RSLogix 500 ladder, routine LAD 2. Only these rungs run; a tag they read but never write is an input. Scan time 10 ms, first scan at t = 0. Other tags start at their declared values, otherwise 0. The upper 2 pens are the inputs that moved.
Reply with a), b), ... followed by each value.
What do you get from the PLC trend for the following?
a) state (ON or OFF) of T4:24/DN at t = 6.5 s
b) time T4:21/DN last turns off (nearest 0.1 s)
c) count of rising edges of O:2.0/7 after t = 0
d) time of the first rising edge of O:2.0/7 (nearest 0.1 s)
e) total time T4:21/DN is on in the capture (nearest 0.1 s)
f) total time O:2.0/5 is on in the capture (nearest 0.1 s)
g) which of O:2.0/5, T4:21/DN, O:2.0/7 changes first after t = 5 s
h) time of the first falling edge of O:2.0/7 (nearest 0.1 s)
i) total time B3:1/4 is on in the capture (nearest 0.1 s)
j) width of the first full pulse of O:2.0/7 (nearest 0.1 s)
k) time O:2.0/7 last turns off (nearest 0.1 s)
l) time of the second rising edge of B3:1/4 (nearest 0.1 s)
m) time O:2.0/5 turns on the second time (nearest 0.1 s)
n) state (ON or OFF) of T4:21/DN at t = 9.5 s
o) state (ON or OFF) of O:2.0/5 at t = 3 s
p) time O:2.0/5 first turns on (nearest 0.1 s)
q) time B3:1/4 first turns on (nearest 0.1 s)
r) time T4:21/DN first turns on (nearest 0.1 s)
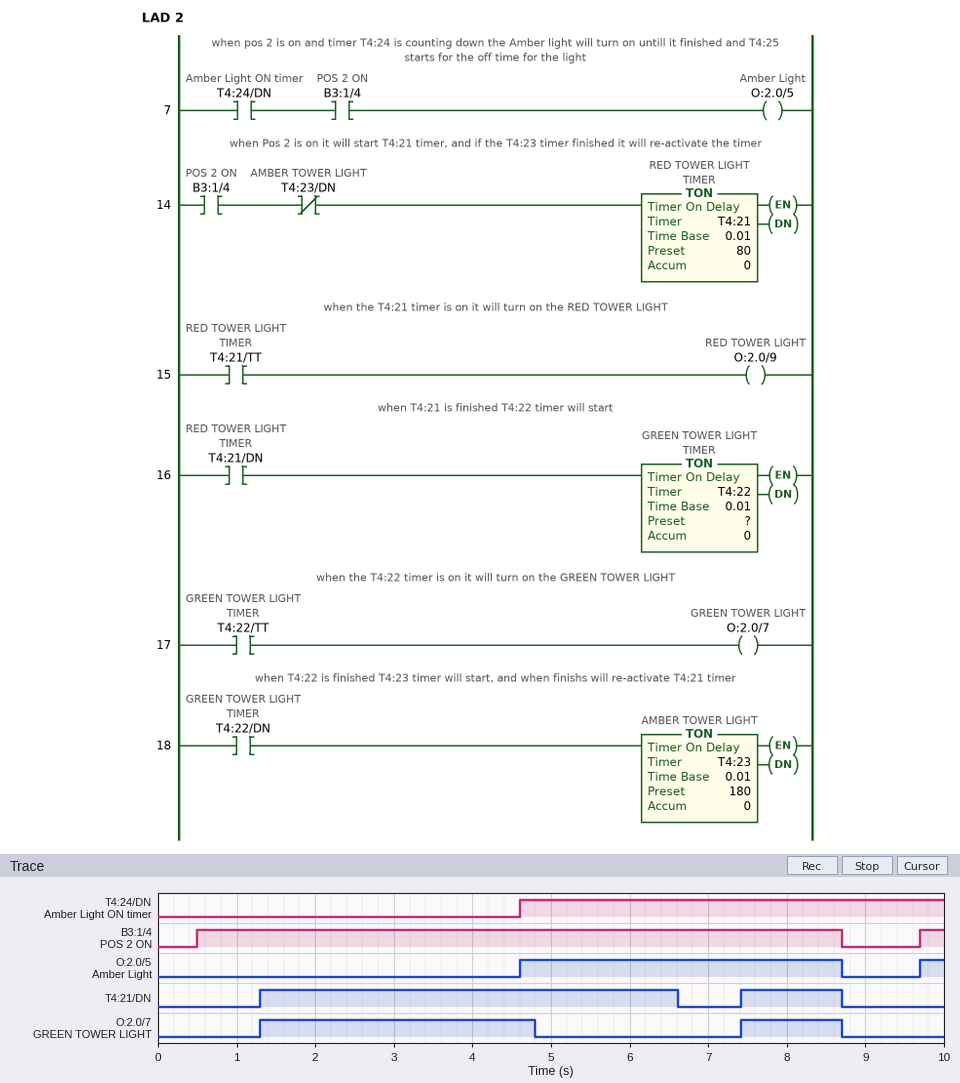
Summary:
a) ON
b) 8.7 s
c) 2
d) 1.3 s
e) 6.6 s
f) 4.4 s
g) T4:21/DN
h) 4.8 s
i) 8.5 s
j) 3.5 s
k) 8.7 s
l) 9.7 s
m) 9.7 s
n) OFF
o) OFF
p) 4.6 s
q) 0.5 s
r) 1.3 s
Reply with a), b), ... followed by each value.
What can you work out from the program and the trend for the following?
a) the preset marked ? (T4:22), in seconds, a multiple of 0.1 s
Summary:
a) 3.5 s
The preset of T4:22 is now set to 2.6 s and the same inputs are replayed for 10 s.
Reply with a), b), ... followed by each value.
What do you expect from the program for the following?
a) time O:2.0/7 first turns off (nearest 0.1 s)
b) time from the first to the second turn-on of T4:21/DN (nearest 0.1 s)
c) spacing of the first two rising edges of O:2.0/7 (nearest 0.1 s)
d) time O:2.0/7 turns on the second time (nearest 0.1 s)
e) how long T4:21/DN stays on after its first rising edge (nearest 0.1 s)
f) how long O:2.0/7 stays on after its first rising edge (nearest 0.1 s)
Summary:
a) 3.9 s
b) 5.2 s
c) 5.2 s
d) 6.5 s
e) 4.4 s
f) 2.6 s
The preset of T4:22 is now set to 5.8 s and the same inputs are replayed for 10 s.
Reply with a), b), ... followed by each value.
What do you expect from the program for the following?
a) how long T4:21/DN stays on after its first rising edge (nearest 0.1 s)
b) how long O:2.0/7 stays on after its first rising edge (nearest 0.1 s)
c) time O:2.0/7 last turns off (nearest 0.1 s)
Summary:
a) 7.4 s
b) 5.8 s
c) 7.1 s
